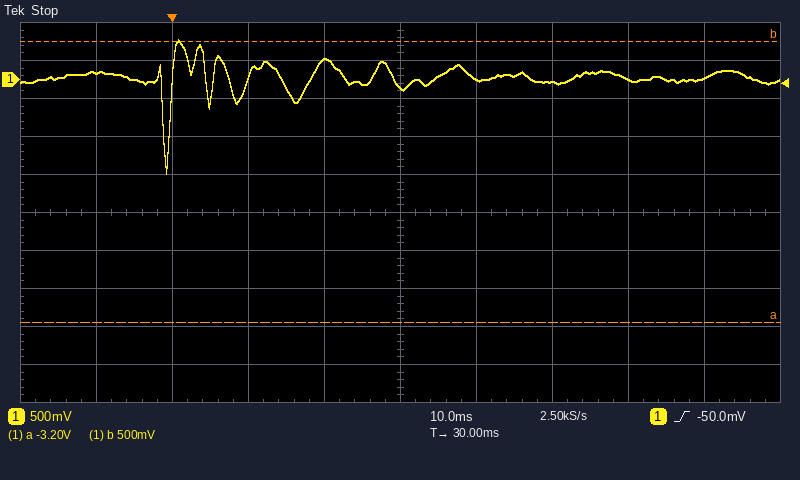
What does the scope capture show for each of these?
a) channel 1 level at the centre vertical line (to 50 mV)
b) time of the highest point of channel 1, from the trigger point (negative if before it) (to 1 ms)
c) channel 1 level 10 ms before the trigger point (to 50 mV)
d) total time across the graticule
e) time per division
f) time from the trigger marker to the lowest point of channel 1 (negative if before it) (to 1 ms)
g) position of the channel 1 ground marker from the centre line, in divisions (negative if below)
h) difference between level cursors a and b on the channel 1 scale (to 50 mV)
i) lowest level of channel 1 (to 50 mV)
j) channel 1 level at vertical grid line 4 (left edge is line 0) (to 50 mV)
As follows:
-100 mV
+1 ms
100 mV
100 ms
10 ms
-1 ms
+3.5 div
3.70 V
-1.25 V
250 mV
